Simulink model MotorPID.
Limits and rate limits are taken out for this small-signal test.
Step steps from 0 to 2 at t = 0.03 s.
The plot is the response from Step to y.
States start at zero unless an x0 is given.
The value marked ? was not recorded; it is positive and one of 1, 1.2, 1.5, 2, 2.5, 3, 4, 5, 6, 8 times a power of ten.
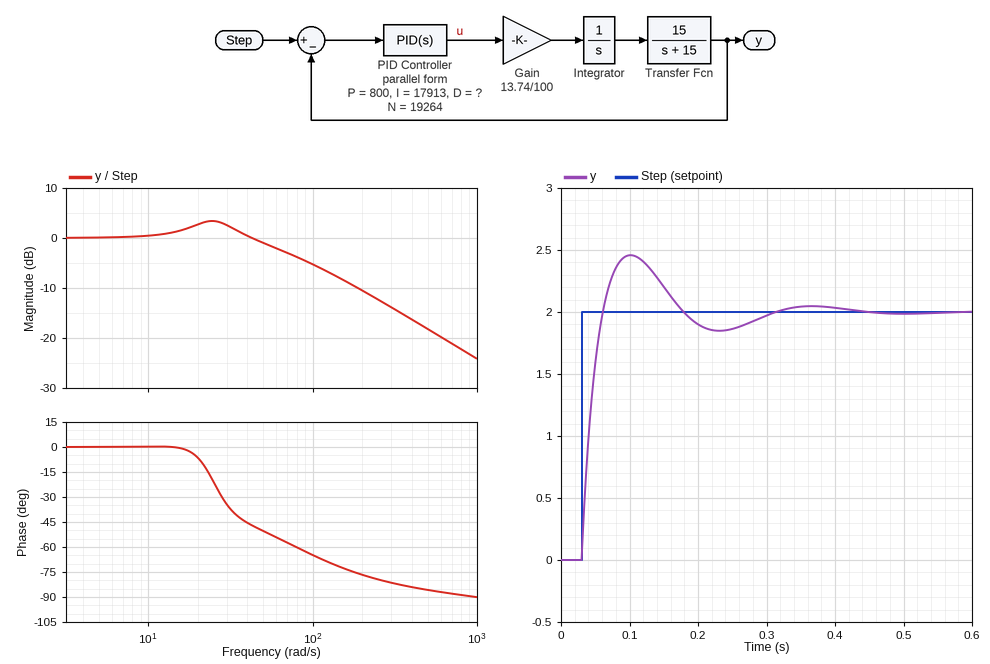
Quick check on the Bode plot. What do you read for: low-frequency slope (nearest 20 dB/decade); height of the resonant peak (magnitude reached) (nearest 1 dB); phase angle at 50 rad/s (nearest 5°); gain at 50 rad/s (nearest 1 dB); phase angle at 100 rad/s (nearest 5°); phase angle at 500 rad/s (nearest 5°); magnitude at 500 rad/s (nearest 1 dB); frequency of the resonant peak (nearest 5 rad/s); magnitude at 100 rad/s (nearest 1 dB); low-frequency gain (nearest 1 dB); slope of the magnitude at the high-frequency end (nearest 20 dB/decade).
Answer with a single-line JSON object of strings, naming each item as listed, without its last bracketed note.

{"low-frequency slope": "0 dB/decade", "height of the resonant peak (magnitude reached)": "3 dB", "phase angle at 50 rad/s": "-50°", "gain at 50 rad/s": "-1 dB", "phase angle at 100 rad/s": "-65°", "phase angle at 500 rad/s": "-85°", "magnitude at 500 rad/s": "-18 dB", "frequency of the resonant peak": "25 rad/s", "magnitude at 100 rad/s": "-5 dB", "low-frequency gain": "0 dB", "slope of the magnitude at the high-frequency end": "-20 dB/decade"}
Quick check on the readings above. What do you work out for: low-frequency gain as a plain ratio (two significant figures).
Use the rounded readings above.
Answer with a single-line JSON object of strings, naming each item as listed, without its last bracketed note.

{"low-frequency gain as a plain ratio": "1.0"}
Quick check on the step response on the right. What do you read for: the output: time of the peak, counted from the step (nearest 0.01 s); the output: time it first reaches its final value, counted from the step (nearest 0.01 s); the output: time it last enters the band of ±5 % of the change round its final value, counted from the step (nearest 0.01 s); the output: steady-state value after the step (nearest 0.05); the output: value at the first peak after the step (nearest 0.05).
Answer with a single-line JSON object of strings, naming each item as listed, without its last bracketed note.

{"the output: time of the peak, counted from the step": "0.07 s", "the output: time it first reaches its final value, counted from the step": "0.03 s", "the output: time it last enters the band of ±5 % of the change round its final value, counted from the step": "0.24 s", "the output: steady-state value after the step": "2.00", "the output: value at the first peak after the step": "2.45"}
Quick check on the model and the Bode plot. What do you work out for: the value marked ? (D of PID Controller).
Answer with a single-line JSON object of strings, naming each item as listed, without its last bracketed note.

{"the value marked ?": "30"}
